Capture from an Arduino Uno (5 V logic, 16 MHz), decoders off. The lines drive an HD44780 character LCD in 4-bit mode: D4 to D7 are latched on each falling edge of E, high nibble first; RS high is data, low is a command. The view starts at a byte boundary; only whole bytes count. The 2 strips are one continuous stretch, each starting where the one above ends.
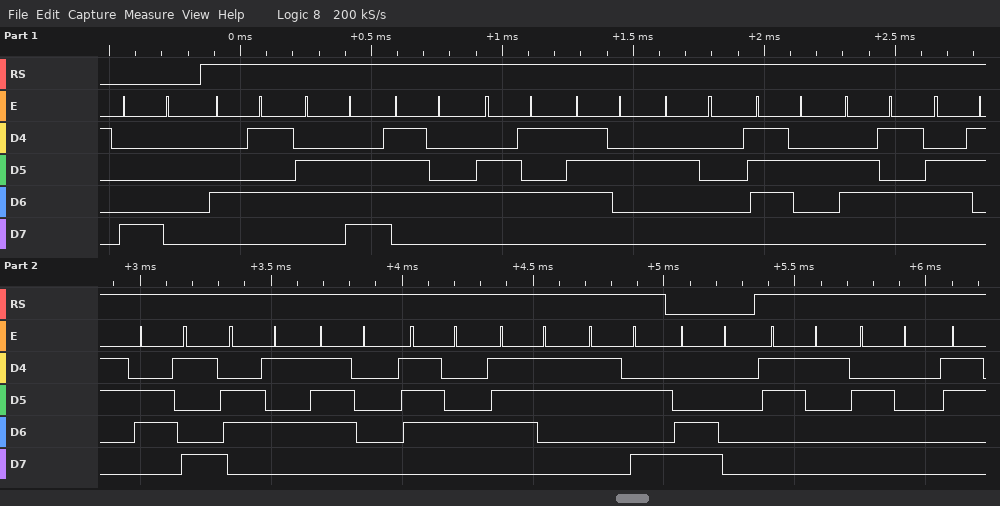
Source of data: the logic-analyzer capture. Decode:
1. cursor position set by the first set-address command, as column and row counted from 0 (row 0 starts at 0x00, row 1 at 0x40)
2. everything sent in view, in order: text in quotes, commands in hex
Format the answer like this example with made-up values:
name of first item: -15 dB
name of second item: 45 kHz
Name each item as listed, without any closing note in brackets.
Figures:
cursor position set by the first set-address command, as column and row counted from 0: column 0, row 0
everything sent in view, in order: text in quotes, commands in hex: 0x80 "Enter reciepts:" 0xC0 "1 "
